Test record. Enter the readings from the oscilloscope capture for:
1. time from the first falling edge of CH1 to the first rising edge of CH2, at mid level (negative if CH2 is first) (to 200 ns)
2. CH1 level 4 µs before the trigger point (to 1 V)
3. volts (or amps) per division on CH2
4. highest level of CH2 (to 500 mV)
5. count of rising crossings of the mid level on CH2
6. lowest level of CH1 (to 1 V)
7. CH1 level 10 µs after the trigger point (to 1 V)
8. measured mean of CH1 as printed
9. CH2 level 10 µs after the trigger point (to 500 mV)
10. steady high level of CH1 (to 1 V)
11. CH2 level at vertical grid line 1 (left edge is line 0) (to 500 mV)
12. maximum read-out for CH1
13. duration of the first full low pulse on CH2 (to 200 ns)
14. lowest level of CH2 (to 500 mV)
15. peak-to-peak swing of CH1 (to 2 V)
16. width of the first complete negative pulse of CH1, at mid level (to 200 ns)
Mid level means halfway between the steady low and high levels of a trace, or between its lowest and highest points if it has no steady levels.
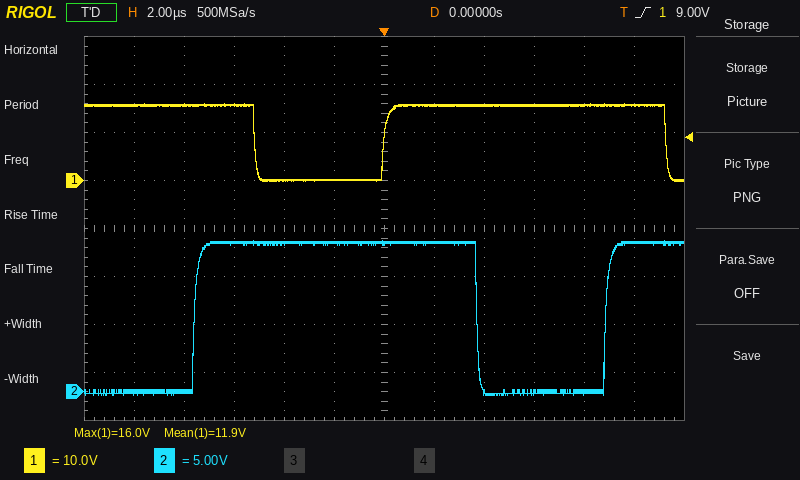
-2.4 µs
0 V
5 V
16.0 V
2
0 V
16 V
11.9 V
15.5 V
16 V
0.0 V
16.0 V
5.2 µs
-500 mV
16 V
5.2 µs
